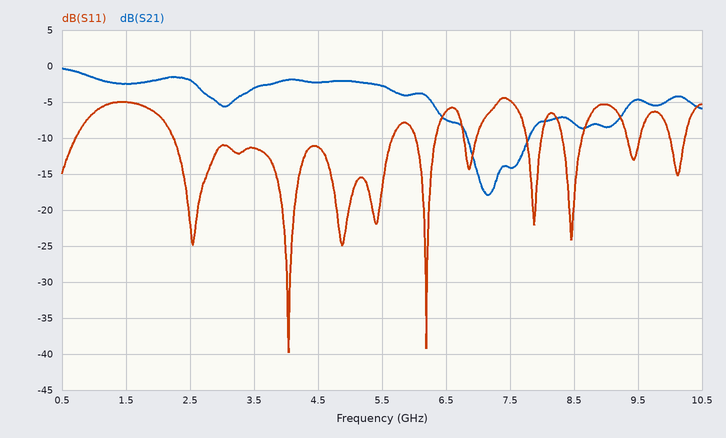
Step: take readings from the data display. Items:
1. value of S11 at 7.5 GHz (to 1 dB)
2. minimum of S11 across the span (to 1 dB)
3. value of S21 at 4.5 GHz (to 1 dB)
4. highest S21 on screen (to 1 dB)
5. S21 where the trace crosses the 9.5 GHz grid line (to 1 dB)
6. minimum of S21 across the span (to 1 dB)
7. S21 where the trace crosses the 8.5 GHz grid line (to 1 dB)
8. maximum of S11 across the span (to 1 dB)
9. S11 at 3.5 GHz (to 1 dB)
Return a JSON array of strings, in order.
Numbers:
["-5 dB", "-40 dB", "-2 dB", "0 dB", "-5 dB", "-18 dB", "-8 dB", "-4 dB", "-11 dB"]
